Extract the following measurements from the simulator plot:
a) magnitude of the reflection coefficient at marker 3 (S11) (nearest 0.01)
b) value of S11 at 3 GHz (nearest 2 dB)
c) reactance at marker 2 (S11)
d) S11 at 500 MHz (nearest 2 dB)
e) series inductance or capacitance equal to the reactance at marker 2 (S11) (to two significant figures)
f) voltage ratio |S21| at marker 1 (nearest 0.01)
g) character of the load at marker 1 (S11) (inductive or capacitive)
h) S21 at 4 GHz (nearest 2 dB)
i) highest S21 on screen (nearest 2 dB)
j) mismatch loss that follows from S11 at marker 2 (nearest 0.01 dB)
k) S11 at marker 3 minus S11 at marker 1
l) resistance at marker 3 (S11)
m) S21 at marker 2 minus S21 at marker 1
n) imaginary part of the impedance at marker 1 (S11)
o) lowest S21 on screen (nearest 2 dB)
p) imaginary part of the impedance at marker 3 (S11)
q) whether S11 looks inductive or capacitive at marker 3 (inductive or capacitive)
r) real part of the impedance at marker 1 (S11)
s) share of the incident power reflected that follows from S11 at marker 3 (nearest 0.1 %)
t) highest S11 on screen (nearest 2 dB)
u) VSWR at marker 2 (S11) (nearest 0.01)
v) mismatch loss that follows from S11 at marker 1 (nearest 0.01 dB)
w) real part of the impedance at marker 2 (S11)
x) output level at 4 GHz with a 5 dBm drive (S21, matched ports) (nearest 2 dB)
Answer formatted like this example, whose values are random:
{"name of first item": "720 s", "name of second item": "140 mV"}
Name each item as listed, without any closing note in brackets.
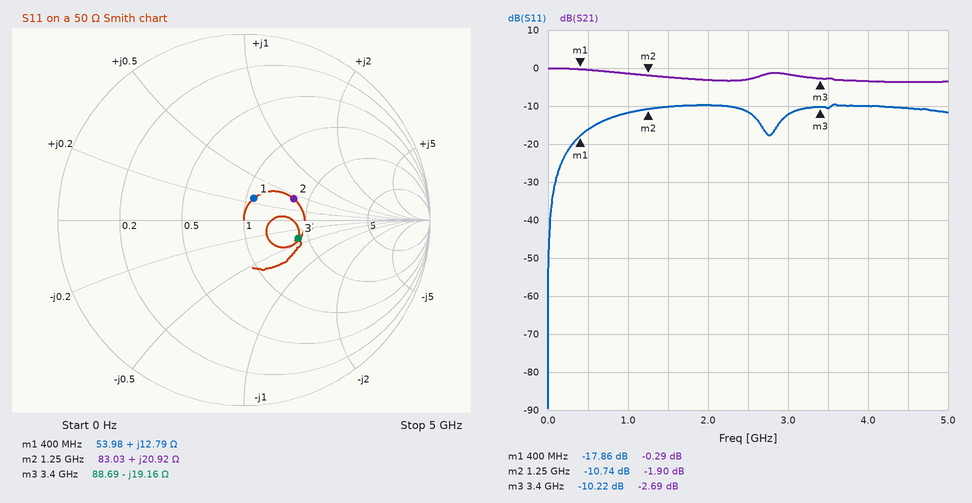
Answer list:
{"magnitude of the reflection coefficient at marker 3 (S11)": "0.31", "value of S11 at 3 GHz": "-12 dB", "reactance at marker 2": "+20.92 Ω", "S11 at 500 MHz": "-16 dB", "series inductance or capacitance equal to the reactance at marker 2 (S11)": "2.7 nH", "voltage ratio |S21| at marker 1": "0.97", "character of the load at marker 1 (S11)": "inductive", "S21 at 4 GHz": "-4 dB", "highest S21 on screen": "0 dB", "mismatch loss that follows from S11 at marker 2": "0.38 dB", "S11 at marker 3 minus S11 at marker 1": "7.64 dB", "resistance at marker 3": "88.69 Ω", "S21 at marker 2 minus S21 at marker 1": "-1.61 dB", "imaginary part of the impedance at marker 1": "+12.79 Ω", "lowest S21 on screen": "-4 dB", "imaginary part of the impedance at marker 3": "-19.16 Ω", "whether S11 looks inductive or capacitive at marker 3": "capacitive", "real part of the impedance at marker 1": "53.98 Ω", "share of the incident power reflected that follows from S11 at marker 3": "9.5 %", "highest S11 on screen": "-10 dB", "VSWR at marker 2 (S11)": "1.82", "mismatch loss that follows from S11 at marker 1": "0.07 dB", "real part of the impedance at marker 2": "83.03 Ω", "output level at 4 GHz with a 5 dBm drive (S21, matched ports)": "2 dBm"}
